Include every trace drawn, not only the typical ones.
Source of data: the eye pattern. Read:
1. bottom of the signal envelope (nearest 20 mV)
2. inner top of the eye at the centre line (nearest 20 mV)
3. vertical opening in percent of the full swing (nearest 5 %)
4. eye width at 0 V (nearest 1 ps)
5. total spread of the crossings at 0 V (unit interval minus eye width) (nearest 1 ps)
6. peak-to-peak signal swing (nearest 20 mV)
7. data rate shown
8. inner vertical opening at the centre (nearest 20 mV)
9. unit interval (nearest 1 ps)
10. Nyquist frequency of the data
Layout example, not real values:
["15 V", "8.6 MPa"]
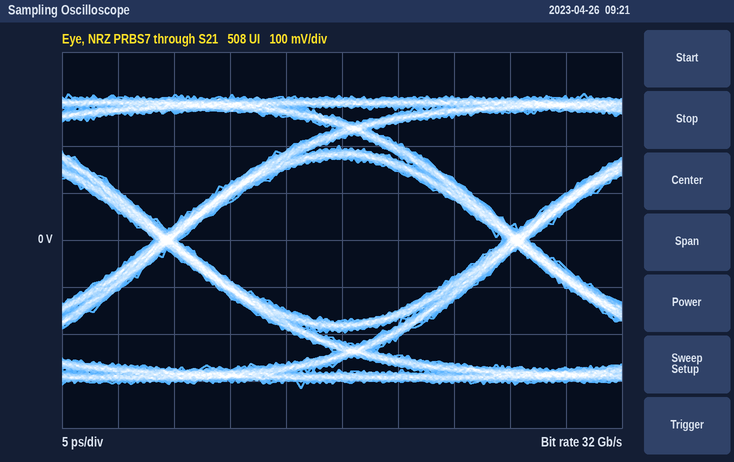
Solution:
["-320 mV", "180 mV", "55 %", "29 ps", "2 ps", "620 mV", "32 Gb/s", "340 mV", "31 ps", "16 GHz"]
